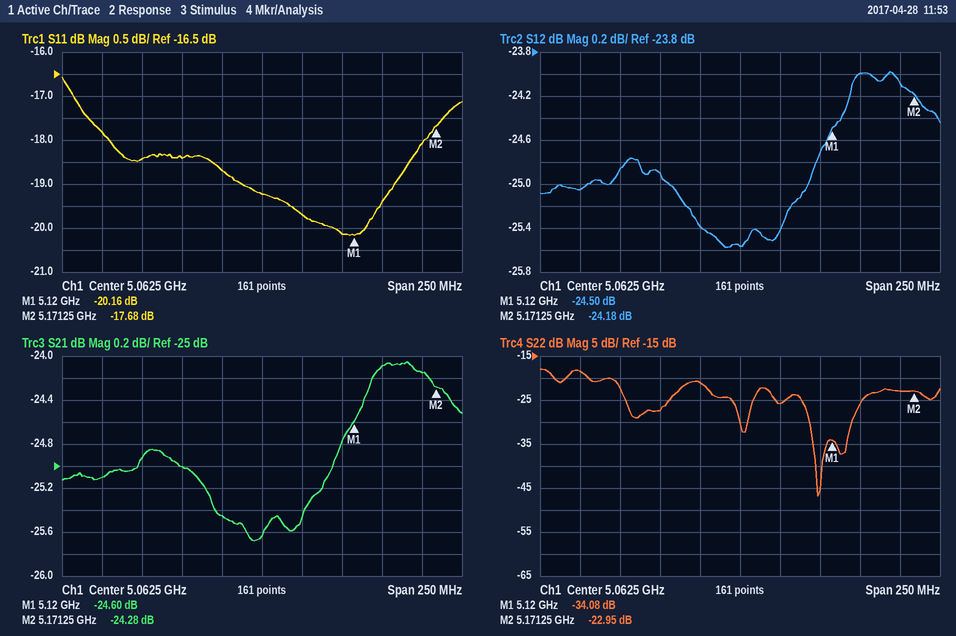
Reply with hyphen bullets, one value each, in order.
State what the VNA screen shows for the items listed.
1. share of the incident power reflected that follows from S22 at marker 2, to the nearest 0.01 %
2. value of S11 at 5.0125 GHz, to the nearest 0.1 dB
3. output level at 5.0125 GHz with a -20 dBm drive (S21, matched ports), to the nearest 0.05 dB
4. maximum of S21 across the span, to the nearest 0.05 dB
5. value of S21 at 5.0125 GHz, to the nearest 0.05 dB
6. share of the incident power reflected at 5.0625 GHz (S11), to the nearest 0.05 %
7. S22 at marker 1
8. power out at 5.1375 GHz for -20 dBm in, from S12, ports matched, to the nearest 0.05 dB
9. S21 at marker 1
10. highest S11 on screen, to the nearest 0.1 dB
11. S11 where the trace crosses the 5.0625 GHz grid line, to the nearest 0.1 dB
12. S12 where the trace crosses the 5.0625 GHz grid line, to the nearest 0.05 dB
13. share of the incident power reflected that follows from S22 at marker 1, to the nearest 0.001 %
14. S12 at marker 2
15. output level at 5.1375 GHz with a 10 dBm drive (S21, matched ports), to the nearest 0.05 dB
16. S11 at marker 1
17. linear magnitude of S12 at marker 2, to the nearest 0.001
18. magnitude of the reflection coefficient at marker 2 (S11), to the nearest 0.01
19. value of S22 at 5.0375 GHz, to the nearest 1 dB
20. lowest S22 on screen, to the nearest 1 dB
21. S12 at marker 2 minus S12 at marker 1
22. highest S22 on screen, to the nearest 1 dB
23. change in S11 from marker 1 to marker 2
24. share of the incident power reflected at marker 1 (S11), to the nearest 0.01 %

- 0.51 %
- -18.4 dB
- -45.00 dBm
- -24.05 dB
- -25.00 dB
- 1.20 %
- -34.08 dB
- -44.00 dBm
- -24.60 dB
- -16.6 dB
- -19.2 dB
- -25.55 dB
- 0.039 %
- -24.18 dB
- -14.10 dBm
- -20.16 dB
- 0.062
- 0.13
- -21 dB
- -47 dB
- 0.32 dB
- -18 dB
- 2.48 dB
- 0.96 %
